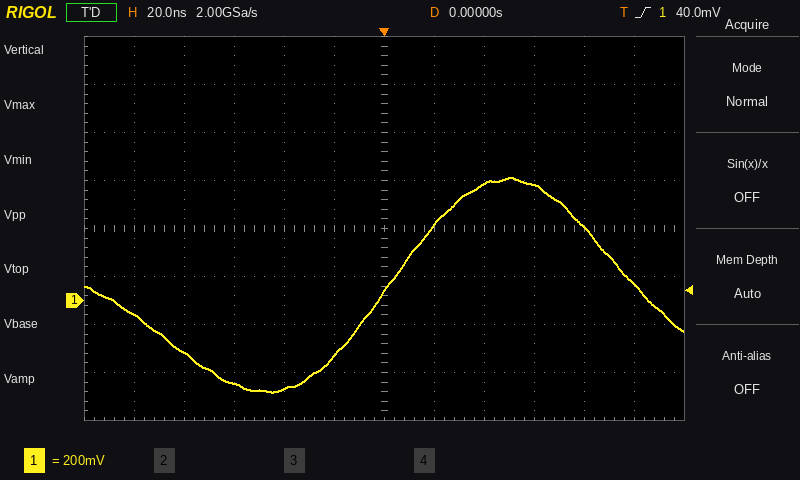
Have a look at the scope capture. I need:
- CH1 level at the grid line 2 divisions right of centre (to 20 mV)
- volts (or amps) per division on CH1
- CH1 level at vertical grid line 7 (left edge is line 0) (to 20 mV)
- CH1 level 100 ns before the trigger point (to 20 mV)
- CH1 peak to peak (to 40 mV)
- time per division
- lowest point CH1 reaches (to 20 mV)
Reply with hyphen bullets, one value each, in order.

- 480 mV
- 200 mV
- 320 mV
- -60 mV
- 880 mV
- 20 ns
- -380 mV
